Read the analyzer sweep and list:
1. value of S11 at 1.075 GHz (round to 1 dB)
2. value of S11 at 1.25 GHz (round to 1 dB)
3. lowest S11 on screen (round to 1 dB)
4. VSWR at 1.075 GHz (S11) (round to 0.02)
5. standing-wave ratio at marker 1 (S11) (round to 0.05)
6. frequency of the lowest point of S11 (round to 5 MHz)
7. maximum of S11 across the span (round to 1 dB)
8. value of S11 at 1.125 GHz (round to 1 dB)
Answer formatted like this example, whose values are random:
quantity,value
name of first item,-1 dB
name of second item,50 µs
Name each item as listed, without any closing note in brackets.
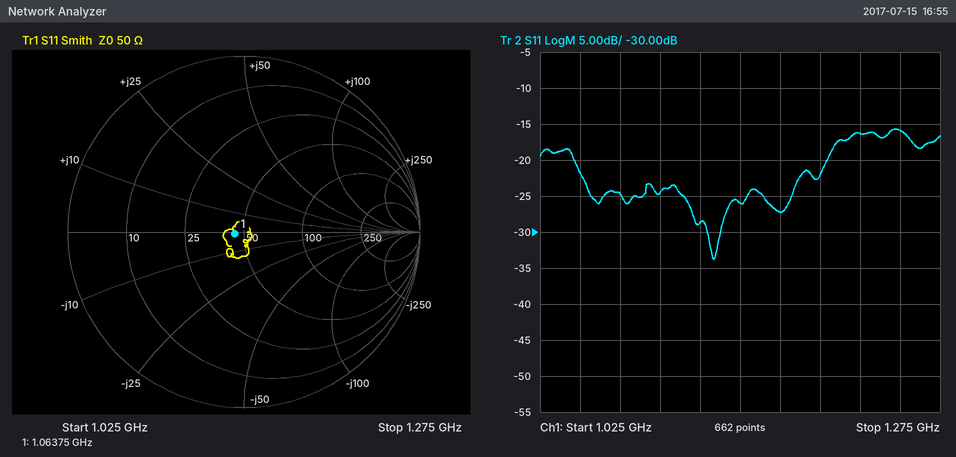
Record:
quantity,value
value of S11 at 1.075 GHz,-25 dB
value of S11 at 1.25 GHz,-16 dB
lowest S11 on screen,-34 dB
VSWR at 1.075 GHz (S11),1.12
standing-wave ratio at marker 1 (S11),1.10
frequency of the lowest point of S11,1.135 GHz
maximum of S11 across the span,-16 dB
value of S11 at 1.125 GHz,-29 dB
